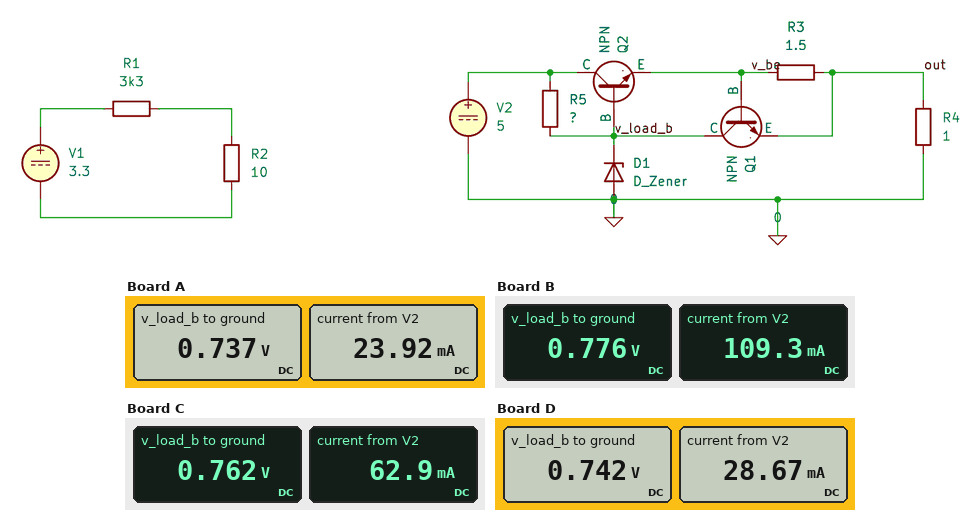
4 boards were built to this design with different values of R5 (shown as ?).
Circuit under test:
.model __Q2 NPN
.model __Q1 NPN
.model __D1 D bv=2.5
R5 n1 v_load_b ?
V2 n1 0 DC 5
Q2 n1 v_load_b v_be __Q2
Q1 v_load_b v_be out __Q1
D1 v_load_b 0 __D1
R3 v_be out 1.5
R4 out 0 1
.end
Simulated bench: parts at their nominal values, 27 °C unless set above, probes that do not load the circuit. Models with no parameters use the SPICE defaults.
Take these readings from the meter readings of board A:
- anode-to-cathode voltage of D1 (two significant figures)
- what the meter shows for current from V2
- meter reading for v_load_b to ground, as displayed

740 mV
23.92 mA
0.737 V
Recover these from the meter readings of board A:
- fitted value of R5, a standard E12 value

180 Ω
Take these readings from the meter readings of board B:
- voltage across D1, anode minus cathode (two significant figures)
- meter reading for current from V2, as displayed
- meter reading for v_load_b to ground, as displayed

780 mV
109.3 mA
0.776 V
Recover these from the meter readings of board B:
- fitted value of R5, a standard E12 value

39 Ω
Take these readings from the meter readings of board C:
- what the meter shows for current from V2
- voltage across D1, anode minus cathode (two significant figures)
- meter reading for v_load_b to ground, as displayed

62.9 mA
760 mV
0.762 V
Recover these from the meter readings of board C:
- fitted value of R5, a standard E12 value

68 Ω
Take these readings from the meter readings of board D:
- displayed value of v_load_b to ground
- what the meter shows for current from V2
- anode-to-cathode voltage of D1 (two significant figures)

0.742 V
28.67 mA
740 mV
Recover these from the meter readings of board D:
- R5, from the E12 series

150 Ω
